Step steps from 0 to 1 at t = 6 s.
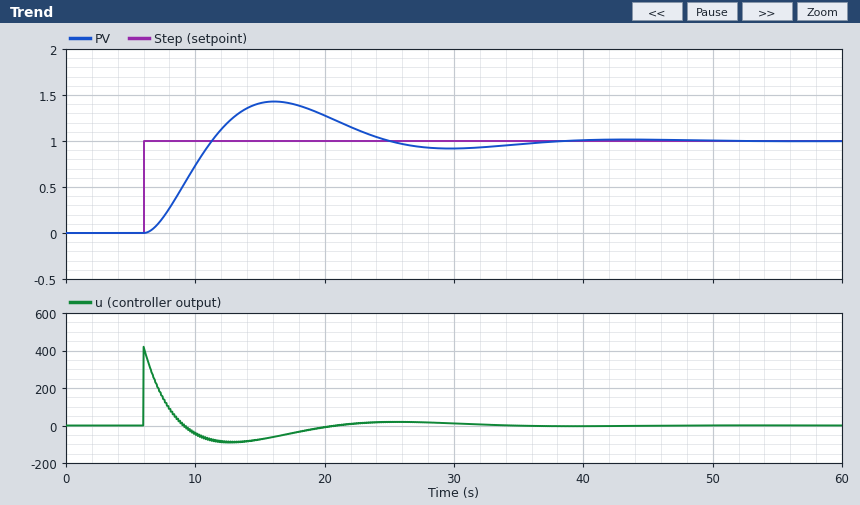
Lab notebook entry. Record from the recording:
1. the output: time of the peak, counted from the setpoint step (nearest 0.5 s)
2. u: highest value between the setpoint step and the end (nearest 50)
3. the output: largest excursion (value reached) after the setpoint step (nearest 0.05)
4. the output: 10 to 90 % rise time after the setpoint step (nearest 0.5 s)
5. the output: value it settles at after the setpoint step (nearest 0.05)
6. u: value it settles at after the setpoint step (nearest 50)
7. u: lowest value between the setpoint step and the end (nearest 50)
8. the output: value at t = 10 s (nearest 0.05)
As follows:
10.0 s
400
1.45
3.5 s
1.00
0
-100
0.75
